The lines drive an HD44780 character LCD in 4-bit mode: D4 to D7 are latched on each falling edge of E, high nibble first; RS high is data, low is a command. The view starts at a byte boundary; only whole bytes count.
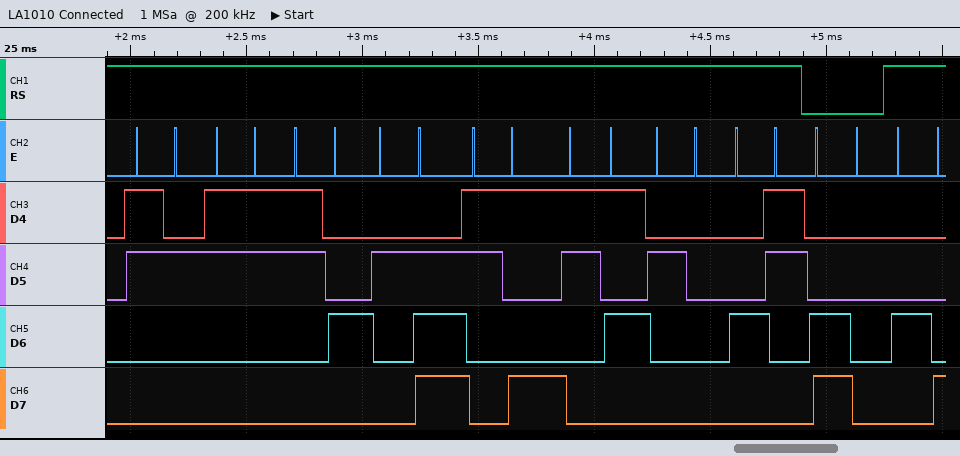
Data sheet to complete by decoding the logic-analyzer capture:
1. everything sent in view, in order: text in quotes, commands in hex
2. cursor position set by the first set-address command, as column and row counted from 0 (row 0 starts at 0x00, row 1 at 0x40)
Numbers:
"234.95 C" 0xC0 "H"
column 0, row 1
